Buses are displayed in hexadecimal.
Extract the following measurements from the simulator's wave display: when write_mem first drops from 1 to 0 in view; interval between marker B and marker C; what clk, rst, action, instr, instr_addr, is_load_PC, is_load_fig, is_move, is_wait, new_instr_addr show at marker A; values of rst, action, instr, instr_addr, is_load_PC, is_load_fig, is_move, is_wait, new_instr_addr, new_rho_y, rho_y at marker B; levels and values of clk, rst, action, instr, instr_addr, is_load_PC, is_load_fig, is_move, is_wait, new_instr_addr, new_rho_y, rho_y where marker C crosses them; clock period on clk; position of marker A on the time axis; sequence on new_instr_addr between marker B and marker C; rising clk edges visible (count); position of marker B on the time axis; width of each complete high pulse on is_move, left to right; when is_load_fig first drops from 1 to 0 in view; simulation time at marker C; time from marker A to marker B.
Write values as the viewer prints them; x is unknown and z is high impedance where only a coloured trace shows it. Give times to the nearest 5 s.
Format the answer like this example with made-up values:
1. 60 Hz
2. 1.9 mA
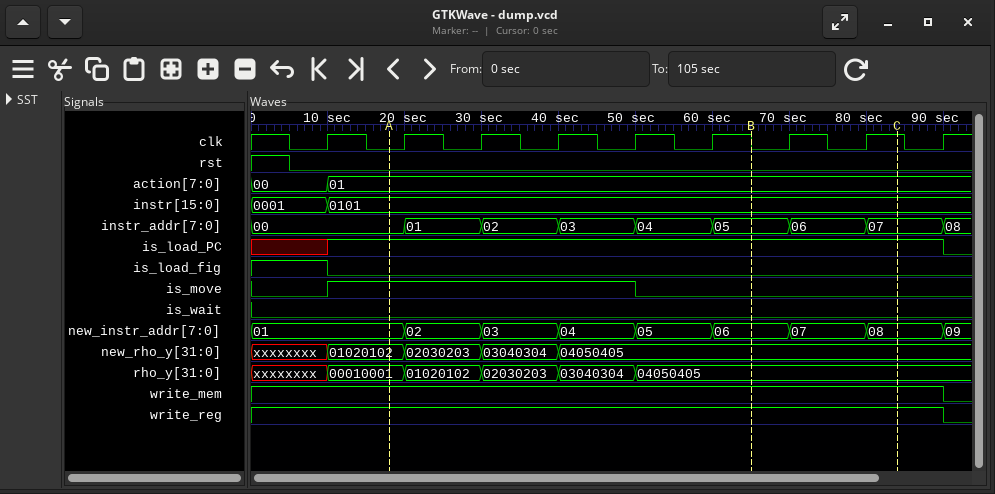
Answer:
1. 90 s
2. 20 s
3. clk=0, rst=0, action=01, instr=0101, instr_addr=00, is_load_PC=1, is_load_fig=0, is_move=1, is_wait=0, new_instr_addr=01
4. rst=0, action=01, instr=0101, instr_addr=05, is_load_PC=1, is_load_fig=0, is_move=0, is_wait=0, new_instr_addr=06, new_rho_y=04050405, rho_y=04050405
5. clk=1, rst=0, action=01, instr=0101, instr_addr=07, is_load_PC=1, is_load_fig=0, is_move=0, is_wait=0, new_instr_addr=08, new_rho_y=04050405, rho_y=04050405
6. 10 s
7. 20 s
8. 06, 07, 08
9. 9
10. 65 s
11. 40 s
12. 10 s
13. 85 s
14. 45 s
